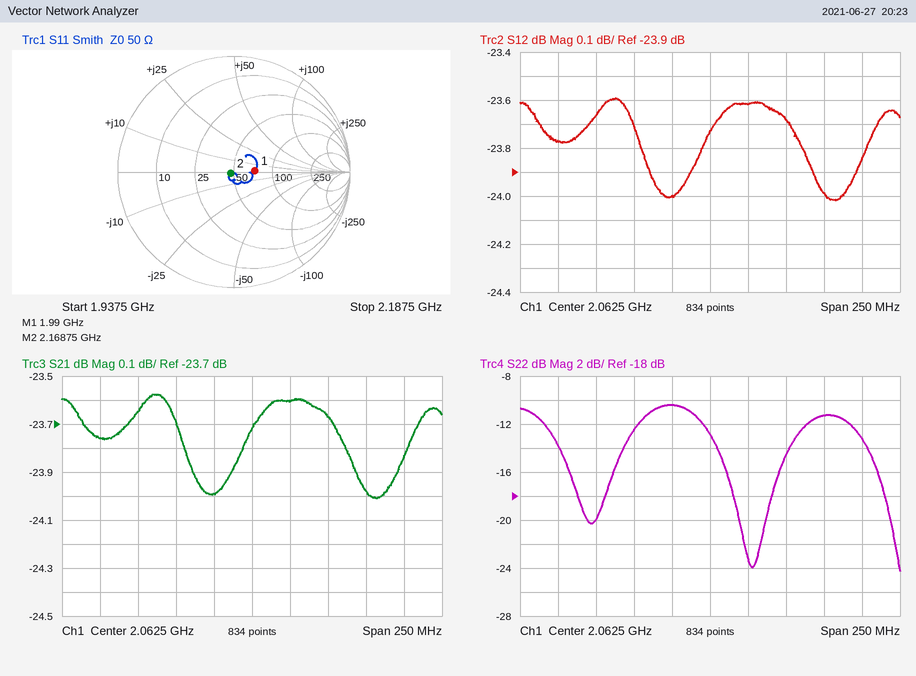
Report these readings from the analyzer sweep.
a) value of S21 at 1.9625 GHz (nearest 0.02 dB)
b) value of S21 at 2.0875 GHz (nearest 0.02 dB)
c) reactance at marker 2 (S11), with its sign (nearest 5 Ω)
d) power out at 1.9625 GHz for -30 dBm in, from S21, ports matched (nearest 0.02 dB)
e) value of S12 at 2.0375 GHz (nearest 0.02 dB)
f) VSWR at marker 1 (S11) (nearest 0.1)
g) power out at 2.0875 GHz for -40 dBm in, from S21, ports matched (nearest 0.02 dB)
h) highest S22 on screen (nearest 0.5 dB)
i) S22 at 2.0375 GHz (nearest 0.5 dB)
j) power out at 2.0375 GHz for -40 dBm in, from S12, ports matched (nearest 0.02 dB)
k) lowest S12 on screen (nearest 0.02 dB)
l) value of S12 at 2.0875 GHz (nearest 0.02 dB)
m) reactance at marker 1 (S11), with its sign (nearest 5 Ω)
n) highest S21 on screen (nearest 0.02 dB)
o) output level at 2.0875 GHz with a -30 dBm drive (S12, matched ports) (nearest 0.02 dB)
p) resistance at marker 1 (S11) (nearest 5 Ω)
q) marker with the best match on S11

-23.76 dB
-23.60 dB
0 Ω
-53.76 dBm
-24.00 dB
1.4
-63.60 dBm
-10.5 dB
-10.5 dB
-64.00 dBm
-24.02 dB
-23.62 dB
0 Ω
-23.58 dB
-53.62 dBm
70 Ω
marker 2
